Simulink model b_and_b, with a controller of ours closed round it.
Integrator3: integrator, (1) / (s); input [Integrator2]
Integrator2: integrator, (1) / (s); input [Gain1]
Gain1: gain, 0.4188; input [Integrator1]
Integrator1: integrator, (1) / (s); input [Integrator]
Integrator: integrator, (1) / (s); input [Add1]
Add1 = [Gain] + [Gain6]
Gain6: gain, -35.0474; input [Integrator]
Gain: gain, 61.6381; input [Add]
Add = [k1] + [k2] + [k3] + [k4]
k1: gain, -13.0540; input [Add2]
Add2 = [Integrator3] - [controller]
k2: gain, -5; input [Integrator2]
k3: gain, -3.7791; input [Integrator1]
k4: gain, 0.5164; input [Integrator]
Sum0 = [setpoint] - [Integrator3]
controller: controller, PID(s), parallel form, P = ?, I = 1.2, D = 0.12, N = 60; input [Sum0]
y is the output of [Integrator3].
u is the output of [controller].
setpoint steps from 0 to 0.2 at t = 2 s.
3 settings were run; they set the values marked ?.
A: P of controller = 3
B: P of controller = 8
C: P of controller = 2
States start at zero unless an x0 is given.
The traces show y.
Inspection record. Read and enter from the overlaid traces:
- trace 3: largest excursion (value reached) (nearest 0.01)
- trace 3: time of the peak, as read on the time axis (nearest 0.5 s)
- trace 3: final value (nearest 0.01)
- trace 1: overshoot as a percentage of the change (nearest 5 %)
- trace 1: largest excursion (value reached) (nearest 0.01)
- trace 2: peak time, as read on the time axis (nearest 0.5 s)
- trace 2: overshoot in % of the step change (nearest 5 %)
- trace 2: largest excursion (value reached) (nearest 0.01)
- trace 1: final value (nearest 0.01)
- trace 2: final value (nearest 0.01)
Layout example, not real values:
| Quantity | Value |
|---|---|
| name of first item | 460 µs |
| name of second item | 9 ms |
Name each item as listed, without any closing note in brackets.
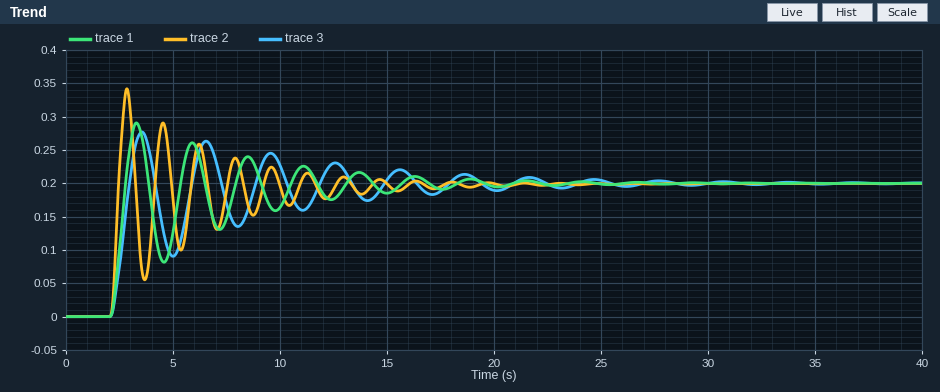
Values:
| Quantity | Value |
|---|---|
| trace 3: largest excursion (value reached) | 0.28 |
| trace 3: time of the peak, as read on the time axis | 3.5 s |
| trace 3: final value | 0.20 |
| trace 1: overshoot as a percentage of the change | 45 % |
| trace 1: largest excursion (value reached) | 0.29 |
| trace 2: peak time, as read on the time axis | 3.0 s |
| trace 2: overshoot in % of the step change | 70 % |
| trace 2: largest excursion (value reached) | 0.34 |
| trace 1: final value | 0.20 |
| trace 2: final value | 0.20 |
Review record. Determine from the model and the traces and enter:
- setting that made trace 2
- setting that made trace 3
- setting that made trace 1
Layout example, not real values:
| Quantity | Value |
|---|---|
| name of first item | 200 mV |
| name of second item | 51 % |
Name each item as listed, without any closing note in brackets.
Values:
| Quantity | Value |
|---|---|
| setting that made trace 2 | B |
| setting that made trace 3 | C |
| setting that made trace 1 | A |
